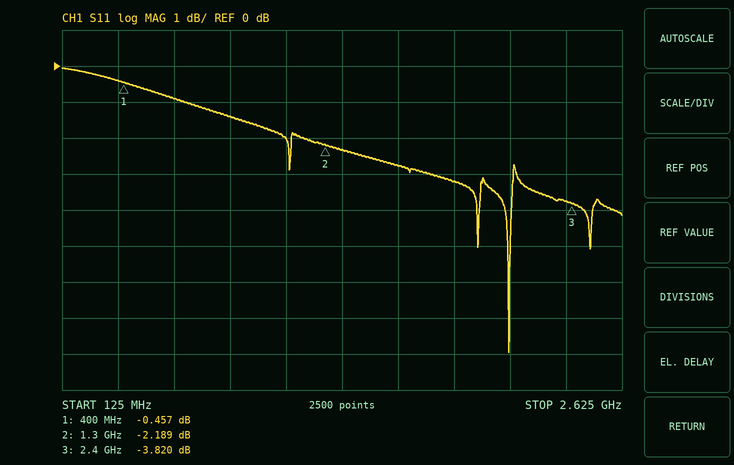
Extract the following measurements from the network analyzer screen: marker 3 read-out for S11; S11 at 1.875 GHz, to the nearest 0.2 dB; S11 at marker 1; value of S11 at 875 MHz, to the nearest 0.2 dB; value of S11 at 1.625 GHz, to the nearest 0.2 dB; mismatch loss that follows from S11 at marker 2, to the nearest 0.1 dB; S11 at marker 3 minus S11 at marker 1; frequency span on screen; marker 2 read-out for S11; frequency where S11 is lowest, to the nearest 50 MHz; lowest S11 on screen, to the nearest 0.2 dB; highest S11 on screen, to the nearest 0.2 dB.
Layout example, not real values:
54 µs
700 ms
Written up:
-3.820 dB
-3.2 dB
-0.457 dB
-1.4 dB
-2.8 dB
4.0 dB
-3.363 dB
2.5 GHz
-2.189 dB
2.10 GHz
-8.0 dB
0.0 dB
